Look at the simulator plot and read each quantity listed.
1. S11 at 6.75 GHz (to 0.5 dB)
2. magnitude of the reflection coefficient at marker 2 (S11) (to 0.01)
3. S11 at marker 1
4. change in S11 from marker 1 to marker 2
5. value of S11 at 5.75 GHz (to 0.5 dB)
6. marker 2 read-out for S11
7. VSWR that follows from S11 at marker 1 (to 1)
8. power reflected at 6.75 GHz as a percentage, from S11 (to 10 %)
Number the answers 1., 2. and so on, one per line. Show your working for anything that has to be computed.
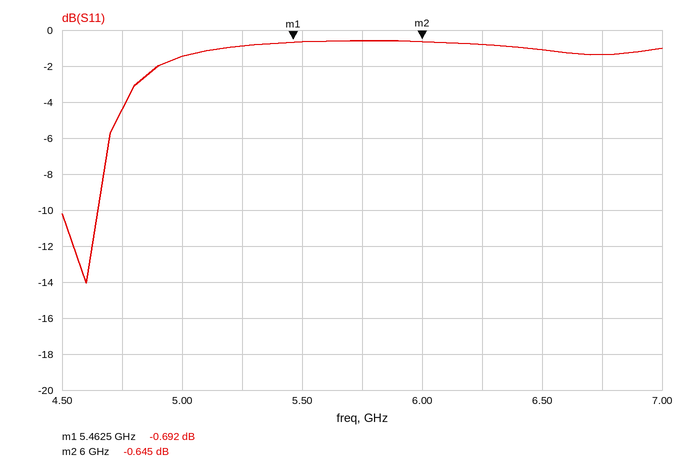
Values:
1. -1.5 dB
2. 10^(-0.645/20) ≈ 0.93
3. -0.692 dB
4. -0.645 − (-0.692) = 0.047 dB
5. -0.5 dB
6. -0.645 dB
7. (1 + 0.9234)/(1 − 0.9234) ≈ 25
8. 10^(-1.5/10) ≈ 70.8 %, so 70 % to the nearest 10 %
